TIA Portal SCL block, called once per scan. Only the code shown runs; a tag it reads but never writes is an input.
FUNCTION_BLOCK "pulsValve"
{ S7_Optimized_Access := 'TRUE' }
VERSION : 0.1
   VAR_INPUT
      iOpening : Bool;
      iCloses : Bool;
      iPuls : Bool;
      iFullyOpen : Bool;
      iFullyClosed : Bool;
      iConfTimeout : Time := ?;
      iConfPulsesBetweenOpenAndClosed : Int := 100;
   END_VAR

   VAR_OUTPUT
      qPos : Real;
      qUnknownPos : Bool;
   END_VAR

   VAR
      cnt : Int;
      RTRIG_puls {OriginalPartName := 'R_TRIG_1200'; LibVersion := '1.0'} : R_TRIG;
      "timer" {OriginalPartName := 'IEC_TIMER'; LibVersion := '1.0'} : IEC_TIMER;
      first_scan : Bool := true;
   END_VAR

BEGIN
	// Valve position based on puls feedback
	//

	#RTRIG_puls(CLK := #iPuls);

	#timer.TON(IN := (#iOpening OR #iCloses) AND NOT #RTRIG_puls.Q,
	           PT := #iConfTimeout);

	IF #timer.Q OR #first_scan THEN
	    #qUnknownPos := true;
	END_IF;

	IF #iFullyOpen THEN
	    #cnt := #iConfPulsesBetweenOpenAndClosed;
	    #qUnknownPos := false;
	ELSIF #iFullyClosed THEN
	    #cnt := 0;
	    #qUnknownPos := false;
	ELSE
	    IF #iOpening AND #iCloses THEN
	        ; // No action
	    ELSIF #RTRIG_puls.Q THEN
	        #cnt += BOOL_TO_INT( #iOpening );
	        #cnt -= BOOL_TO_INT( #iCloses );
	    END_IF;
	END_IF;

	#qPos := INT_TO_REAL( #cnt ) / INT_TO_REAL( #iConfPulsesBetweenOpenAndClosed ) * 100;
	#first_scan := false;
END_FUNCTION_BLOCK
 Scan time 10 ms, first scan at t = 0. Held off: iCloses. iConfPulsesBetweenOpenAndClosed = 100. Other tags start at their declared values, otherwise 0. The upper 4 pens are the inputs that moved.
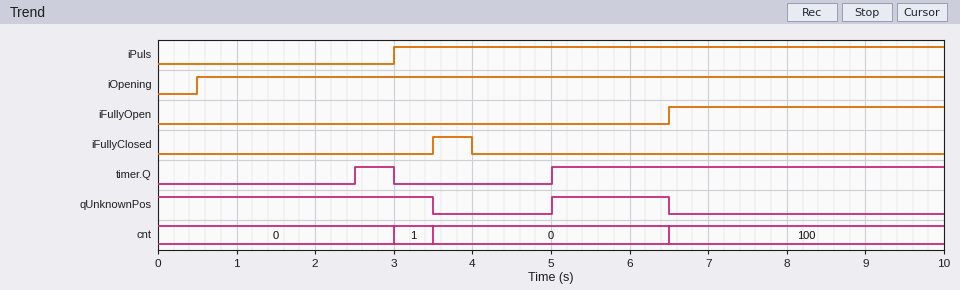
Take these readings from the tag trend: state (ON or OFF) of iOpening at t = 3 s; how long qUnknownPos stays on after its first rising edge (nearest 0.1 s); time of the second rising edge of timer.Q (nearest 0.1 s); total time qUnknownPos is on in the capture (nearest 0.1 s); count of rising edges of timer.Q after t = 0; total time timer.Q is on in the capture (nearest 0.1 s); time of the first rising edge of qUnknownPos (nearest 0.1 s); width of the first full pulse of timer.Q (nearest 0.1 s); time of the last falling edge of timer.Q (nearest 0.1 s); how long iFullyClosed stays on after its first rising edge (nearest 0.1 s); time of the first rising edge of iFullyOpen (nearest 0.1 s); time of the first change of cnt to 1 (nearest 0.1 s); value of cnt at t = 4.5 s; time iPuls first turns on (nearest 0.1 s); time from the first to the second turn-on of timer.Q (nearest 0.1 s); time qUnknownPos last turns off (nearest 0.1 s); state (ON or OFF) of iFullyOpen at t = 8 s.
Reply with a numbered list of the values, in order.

1. ON
2. 1.5 s
3. 5.0 s
4. 5.0 s
5. 2
6. 5.5 s
7. 5.0 s
8. 0.5 s
9. 3.0 s
10. 0.5 s
11. 6.5 s
12. 3.0 s
13. 0
14. 3.0 s
15. 2.5 s
16. 6.5 s
17. ON
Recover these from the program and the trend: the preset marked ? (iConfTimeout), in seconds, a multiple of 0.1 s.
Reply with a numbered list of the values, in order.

1. 2.0 s
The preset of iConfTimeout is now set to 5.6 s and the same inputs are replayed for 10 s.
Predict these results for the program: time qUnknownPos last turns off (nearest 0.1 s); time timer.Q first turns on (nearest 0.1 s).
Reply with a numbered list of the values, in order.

1. 3.5 s
2. 8.6 s
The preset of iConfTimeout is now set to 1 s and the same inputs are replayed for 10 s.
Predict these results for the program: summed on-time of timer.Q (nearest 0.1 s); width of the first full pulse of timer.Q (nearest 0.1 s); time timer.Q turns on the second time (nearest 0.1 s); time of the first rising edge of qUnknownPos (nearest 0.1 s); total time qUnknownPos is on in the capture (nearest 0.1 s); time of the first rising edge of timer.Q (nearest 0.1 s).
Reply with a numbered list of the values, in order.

1. 7.5 s
2. 1.5 s
3. 4.0 s
4. 4.0 s
5. 6.0 s
6. 1.5 s
